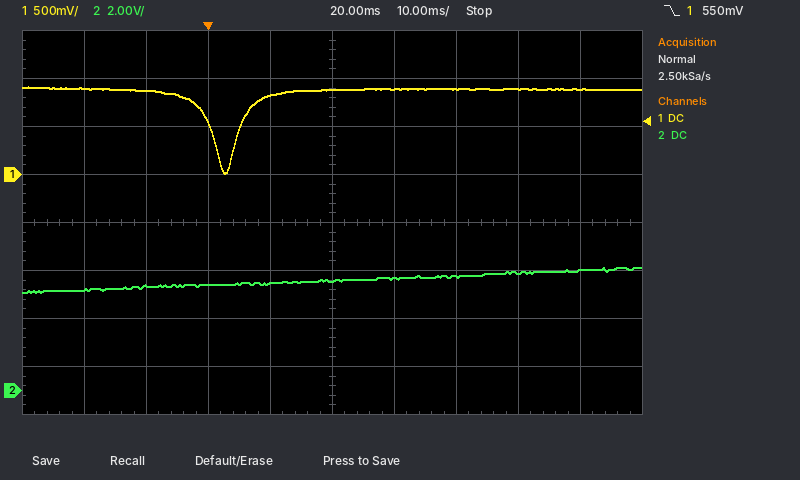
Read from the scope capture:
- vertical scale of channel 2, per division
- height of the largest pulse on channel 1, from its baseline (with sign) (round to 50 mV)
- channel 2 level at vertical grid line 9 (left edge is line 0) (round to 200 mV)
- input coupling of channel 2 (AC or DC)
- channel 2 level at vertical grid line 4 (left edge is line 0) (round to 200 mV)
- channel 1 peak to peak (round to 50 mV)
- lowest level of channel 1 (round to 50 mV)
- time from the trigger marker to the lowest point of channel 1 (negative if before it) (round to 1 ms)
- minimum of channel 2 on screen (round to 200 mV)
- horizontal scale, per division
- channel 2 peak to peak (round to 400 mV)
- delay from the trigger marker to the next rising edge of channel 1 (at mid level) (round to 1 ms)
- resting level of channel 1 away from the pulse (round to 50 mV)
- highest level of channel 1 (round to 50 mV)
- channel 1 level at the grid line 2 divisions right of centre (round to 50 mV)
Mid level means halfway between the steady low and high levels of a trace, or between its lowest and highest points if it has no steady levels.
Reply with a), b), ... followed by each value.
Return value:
a) 2 V
b) -900 mV
c) 5.0 V
d) DC
e) 4.4 V
f) 900 mV
g) 0 mV
h) +3 ms
i) 4.0 V
j) 10 ms
k) 1.2 V
l) 5 ms
m) 900 mV
n) 900 mV
o) 900 mV
